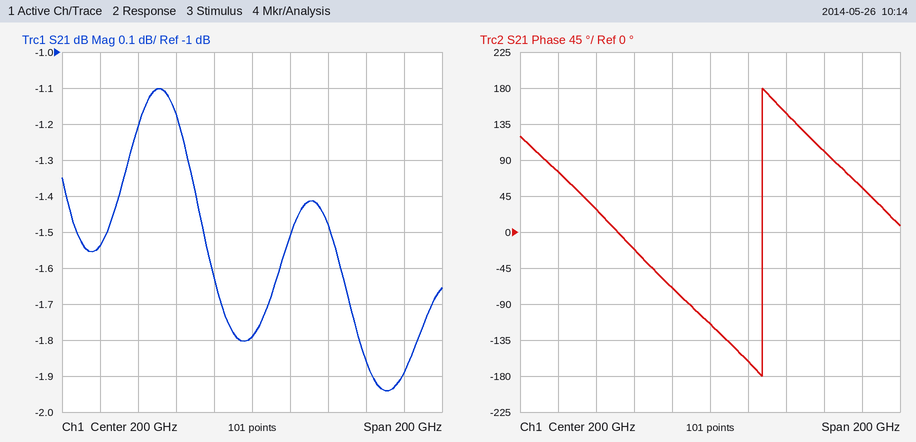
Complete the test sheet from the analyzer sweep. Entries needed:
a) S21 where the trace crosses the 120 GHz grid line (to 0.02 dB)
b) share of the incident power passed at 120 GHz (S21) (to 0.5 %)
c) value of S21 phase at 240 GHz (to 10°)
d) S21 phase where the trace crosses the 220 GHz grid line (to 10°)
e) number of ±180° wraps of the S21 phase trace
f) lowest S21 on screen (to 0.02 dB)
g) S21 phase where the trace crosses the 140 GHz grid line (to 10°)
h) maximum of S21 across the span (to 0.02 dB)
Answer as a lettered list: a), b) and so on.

a) -1.54 dB
b) 70.0 %
c) 150°
d) -160°
e) 1
f) -1.94 dB
g) 30°
h) -1.10 dB
